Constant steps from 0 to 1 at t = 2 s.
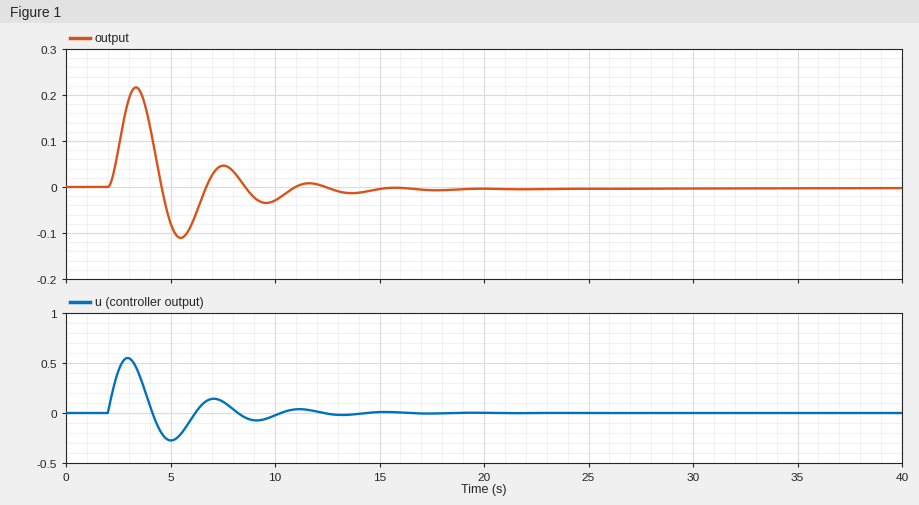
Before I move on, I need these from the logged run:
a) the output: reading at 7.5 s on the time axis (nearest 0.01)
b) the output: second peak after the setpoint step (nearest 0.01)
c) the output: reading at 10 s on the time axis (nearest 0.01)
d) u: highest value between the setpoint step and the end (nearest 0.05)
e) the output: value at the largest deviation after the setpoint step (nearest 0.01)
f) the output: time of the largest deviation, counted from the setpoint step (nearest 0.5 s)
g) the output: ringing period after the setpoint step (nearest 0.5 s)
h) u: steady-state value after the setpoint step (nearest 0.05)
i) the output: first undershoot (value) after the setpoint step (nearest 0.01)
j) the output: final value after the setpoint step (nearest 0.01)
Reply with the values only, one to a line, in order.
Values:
0.05
0.05
-0.03
0.55
0.22
1.5 s
4.0 s
0.00
-0.11
0.00
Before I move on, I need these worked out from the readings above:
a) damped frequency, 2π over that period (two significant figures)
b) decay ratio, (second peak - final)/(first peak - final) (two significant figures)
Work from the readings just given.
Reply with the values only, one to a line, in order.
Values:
1.6 rad/s
0.23
